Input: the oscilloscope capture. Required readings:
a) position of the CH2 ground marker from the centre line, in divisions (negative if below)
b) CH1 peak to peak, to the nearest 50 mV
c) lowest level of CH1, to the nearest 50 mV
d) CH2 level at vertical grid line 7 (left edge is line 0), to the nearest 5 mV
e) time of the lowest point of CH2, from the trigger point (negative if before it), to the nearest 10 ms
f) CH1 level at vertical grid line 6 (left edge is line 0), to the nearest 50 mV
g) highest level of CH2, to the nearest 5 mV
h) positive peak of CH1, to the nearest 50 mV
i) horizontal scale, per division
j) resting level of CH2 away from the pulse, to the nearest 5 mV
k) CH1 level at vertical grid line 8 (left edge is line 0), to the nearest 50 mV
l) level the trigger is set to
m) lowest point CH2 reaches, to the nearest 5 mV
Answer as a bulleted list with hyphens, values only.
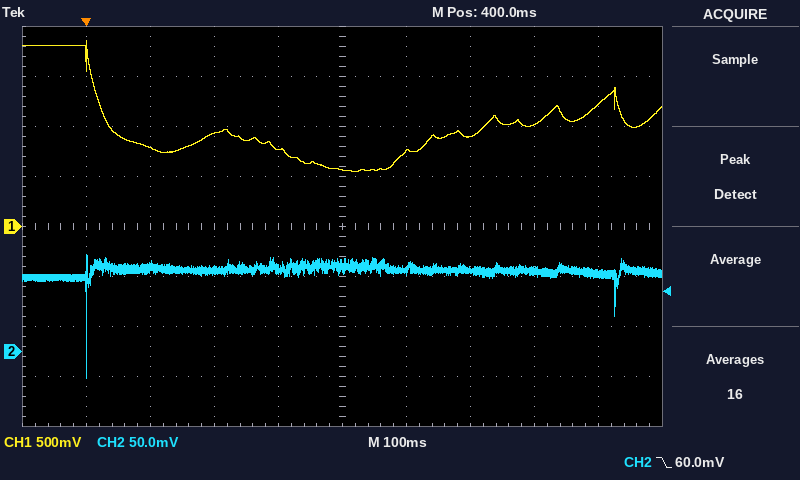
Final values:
- -2.5 div
- 1.30 V
- 550 mV
- 80 mV
- 0 ms
- 750 mV
- 95 mV
- 1.85 V
- 100 ms
- 80 mV
- 1.00 V
- 60.0 mV
- -25 mV
